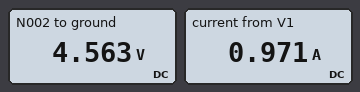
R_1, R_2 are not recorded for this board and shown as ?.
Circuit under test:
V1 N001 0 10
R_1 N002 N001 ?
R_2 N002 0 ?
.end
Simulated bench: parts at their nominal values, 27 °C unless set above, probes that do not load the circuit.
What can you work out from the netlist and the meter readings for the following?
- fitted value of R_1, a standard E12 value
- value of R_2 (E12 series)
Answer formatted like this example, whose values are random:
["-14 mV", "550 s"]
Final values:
["5.6 Ω", "4.7 Ω"]
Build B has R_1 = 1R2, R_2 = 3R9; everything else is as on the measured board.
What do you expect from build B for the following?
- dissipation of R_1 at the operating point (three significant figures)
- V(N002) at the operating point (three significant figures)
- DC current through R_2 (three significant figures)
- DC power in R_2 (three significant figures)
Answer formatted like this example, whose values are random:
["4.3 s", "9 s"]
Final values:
["4.61 W", "7.65 V", "1.96 A", "15.0 W"]
